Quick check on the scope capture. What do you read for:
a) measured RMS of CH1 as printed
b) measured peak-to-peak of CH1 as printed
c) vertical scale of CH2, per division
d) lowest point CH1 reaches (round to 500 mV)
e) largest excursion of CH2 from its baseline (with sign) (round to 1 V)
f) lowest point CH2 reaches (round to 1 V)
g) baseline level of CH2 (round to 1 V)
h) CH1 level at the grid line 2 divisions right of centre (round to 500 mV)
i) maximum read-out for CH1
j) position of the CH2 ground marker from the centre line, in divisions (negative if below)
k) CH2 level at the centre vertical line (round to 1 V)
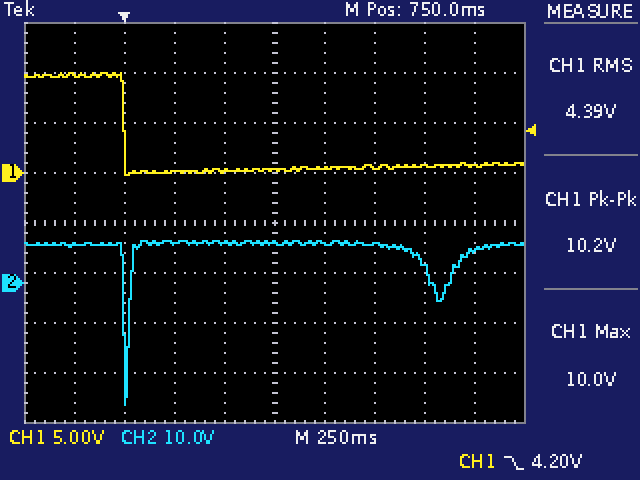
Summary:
4.39 V
10.2 V
10 V
0.0 V
-32 V
-24 V
8 V
500 mV
10.0 V
-1.2 div
8 V
